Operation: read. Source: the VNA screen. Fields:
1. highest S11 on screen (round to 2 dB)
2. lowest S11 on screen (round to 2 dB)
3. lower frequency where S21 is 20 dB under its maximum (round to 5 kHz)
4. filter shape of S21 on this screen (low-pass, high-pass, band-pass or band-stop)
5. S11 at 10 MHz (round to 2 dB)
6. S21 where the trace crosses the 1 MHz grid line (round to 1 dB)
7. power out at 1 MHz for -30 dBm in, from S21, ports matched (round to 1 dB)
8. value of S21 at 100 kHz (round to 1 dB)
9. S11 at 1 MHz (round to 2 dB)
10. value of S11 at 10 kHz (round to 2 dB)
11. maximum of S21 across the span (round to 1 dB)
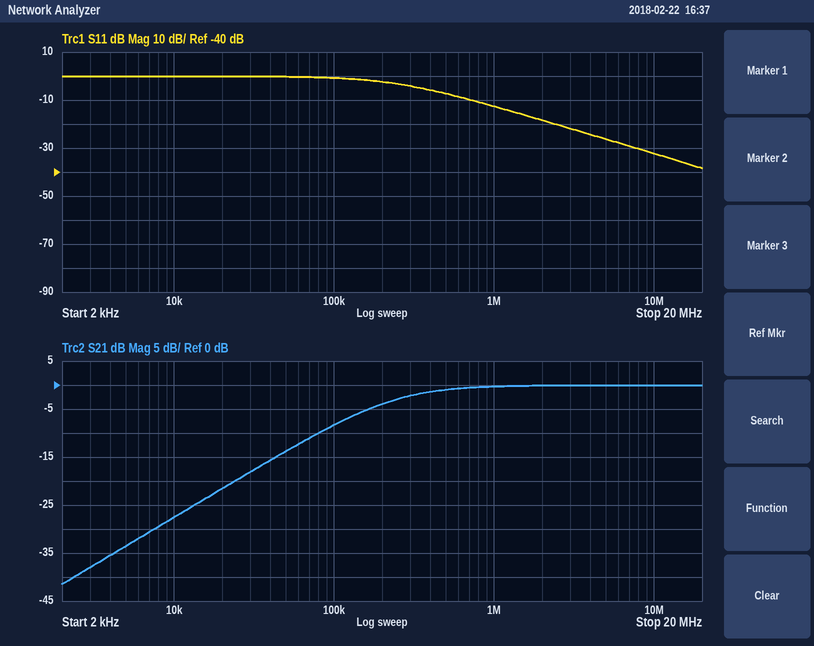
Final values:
0 dB
-38 dB
25 kHz
high-pass
-32 dB
0 dB
-30 dBm
-8 dB
-12 dB
0 dB
0 dB
